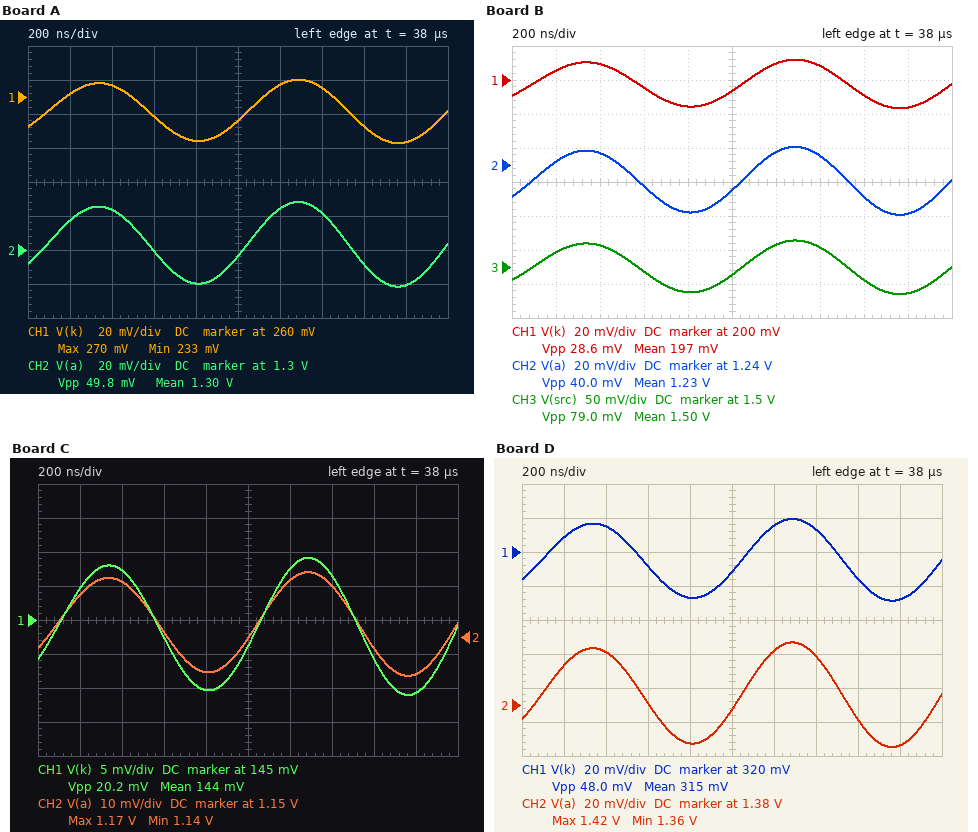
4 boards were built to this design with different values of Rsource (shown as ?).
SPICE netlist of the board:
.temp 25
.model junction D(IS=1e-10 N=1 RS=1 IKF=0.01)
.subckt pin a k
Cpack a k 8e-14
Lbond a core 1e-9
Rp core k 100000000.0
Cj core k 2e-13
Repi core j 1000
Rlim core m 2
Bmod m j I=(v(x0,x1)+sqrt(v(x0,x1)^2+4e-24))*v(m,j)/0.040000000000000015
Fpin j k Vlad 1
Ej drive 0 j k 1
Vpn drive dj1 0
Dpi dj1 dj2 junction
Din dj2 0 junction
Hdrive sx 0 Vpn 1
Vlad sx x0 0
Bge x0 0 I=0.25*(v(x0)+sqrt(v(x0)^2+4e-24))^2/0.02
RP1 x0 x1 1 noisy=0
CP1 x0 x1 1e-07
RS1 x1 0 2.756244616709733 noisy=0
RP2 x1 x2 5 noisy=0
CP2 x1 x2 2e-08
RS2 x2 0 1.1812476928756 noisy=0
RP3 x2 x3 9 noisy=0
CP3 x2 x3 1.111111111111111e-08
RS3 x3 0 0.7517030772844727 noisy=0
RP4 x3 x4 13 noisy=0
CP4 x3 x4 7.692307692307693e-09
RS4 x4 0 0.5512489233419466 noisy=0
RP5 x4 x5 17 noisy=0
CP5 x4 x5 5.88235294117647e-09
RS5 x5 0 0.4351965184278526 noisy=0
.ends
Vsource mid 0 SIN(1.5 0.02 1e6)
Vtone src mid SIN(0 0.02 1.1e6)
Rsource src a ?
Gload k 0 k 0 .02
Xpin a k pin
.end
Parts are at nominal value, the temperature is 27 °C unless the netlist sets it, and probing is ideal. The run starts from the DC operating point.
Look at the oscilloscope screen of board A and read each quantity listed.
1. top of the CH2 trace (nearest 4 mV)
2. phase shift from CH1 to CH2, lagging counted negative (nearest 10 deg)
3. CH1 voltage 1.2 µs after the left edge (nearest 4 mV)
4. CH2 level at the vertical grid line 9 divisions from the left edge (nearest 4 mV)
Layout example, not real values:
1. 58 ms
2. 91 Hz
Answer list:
1. 1.328 V
2. 0 deg
3. 268 mV
4. 1.280 V
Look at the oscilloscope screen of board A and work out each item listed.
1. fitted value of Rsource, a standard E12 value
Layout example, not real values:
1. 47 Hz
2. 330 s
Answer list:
1. 39 Ω
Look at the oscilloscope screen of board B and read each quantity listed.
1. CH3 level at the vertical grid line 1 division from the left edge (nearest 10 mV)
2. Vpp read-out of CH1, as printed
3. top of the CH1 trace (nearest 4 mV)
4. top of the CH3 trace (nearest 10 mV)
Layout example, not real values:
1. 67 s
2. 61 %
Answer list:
1. 1.52 V
2. 28.6 mV
3. 212 mV
4. 1.54 V
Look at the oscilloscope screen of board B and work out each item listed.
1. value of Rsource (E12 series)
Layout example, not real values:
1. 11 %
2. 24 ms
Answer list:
1. 68 Ω
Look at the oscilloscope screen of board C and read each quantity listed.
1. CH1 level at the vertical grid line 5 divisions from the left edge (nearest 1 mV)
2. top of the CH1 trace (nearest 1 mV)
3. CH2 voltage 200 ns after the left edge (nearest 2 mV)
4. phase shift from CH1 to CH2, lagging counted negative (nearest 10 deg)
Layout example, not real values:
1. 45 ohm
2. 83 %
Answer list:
1. 141 mV
2. 154 mV
3. 1.162 V
4. 0 deg
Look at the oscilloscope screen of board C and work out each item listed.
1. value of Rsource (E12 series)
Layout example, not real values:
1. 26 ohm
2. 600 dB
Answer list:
1. 120 Ω
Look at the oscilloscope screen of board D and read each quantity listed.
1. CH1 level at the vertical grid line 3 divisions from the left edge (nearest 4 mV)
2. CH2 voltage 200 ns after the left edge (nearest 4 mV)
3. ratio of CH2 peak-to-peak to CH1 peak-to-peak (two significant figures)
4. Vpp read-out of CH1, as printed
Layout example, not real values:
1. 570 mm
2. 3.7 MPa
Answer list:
1. 312 mV
2. 1.404 V
3. 1.3
4. 48.0 mV
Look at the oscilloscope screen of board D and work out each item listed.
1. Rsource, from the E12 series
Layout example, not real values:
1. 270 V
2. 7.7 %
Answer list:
1. 18 Ω
